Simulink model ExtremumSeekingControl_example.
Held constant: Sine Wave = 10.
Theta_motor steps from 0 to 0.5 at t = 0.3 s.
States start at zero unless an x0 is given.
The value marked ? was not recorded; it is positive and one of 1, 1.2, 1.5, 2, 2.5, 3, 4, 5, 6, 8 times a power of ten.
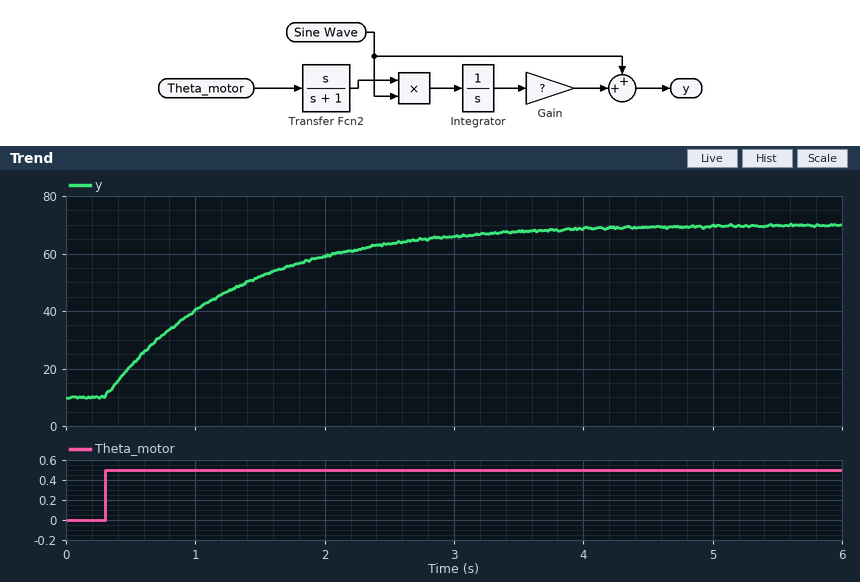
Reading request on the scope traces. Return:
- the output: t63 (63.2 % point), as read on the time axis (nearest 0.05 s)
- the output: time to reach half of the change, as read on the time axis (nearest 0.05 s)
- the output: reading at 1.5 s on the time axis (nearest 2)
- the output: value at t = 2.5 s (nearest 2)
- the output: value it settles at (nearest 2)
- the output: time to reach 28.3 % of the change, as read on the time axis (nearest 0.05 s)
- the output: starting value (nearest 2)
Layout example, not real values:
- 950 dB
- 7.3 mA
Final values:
- 1.30 s
- 1.00 s
- 52
- 64
- 70
- 0.65 s
- 10
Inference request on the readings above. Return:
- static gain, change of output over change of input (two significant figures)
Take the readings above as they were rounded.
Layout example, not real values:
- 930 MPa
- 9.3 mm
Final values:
- 120
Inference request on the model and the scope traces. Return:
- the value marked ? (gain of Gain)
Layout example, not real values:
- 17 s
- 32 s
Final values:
- 12
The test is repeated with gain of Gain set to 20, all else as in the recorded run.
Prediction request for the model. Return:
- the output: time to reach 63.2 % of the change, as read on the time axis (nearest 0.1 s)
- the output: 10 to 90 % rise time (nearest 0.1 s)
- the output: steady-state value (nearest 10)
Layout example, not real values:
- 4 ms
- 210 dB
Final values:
- 1.3 s
- 2.2 s
- 110
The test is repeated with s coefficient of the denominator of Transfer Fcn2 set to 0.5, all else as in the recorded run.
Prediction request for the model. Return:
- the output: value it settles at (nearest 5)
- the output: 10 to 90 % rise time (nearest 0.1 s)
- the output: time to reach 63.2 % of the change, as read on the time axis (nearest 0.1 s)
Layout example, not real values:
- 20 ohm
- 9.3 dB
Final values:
- 70
- 1.1 s
- 0.8 s
